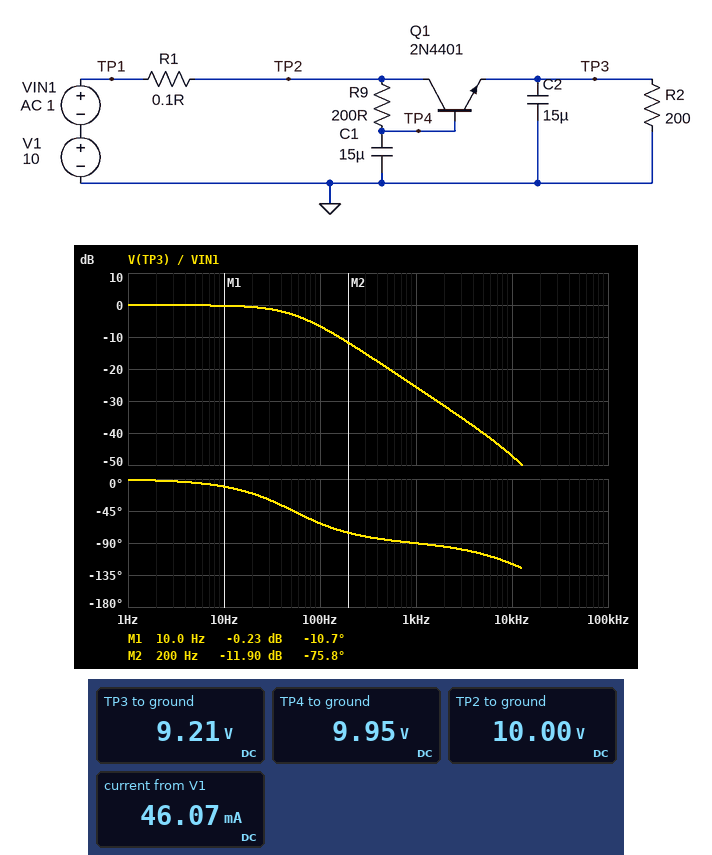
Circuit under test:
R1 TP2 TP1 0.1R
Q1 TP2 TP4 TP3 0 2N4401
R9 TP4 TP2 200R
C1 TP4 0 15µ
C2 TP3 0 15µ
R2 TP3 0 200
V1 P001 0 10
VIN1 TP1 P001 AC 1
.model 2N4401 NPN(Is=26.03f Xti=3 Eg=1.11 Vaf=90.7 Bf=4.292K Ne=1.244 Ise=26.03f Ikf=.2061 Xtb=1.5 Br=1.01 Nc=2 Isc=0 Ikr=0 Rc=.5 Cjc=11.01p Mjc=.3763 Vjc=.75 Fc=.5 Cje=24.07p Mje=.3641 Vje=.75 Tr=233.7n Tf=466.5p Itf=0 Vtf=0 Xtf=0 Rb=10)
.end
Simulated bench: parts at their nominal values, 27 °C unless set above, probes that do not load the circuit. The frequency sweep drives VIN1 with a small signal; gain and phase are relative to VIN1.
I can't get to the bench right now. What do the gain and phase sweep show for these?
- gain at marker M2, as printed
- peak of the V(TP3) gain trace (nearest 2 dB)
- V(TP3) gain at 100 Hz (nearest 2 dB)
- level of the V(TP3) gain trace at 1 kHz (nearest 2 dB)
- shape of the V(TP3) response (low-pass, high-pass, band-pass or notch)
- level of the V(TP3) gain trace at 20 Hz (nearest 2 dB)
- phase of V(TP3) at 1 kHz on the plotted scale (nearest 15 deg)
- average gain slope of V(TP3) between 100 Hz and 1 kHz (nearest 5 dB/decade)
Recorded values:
-11.90 dB
0 dB
-6 dB
-26 dB
low-pass
0 dB
-90 deg
-20 dB/decade
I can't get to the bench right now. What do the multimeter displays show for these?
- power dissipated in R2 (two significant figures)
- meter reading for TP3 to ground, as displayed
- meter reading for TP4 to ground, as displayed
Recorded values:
420 mW
9.21 V
9.95 V
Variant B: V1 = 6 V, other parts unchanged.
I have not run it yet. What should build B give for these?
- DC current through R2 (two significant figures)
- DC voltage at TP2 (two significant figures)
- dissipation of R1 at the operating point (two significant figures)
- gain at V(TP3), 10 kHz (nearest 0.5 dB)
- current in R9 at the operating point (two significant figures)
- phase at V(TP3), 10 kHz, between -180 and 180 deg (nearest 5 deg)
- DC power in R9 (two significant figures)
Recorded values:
26 mA
6.0 V
69 µW
-49.0 dB
130 µA
-135 deg
3.6 µW
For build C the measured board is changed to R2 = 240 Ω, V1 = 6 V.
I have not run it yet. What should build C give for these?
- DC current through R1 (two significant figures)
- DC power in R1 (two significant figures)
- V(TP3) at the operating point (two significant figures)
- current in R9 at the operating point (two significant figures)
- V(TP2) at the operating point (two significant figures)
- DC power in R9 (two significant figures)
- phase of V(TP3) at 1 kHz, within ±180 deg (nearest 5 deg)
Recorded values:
22 mA
48 µW
5.3 V
110 µA
6.0 V
2.6 µW
-95 deg
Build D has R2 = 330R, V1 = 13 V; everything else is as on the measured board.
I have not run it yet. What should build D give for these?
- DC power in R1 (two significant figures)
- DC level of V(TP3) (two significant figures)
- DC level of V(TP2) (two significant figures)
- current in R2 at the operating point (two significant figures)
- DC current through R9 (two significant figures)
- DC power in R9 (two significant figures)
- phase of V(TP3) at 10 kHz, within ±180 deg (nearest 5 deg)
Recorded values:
140 µW
12 V
13 V
37 mA
180 µA
6.8 µW
-125 deg
